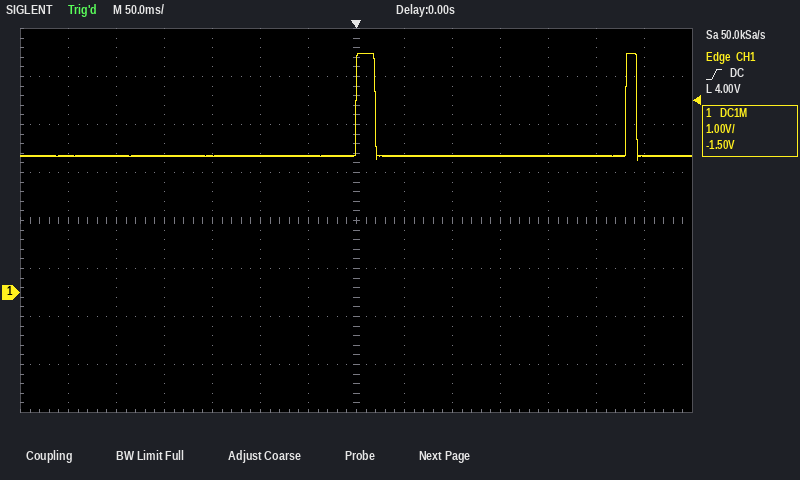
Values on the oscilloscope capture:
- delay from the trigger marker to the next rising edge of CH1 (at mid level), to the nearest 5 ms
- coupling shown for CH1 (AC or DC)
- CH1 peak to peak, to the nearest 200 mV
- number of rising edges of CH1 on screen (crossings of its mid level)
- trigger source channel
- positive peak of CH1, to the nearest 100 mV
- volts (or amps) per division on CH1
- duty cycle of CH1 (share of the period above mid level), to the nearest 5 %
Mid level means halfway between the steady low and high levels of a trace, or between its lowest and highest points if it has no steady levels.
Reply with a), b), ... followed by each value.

a) 280 ms
b) DC
c) 2.2 V
d) 2
e) CH1
f) 5.0 V
g) 1 V
h) 5 %
